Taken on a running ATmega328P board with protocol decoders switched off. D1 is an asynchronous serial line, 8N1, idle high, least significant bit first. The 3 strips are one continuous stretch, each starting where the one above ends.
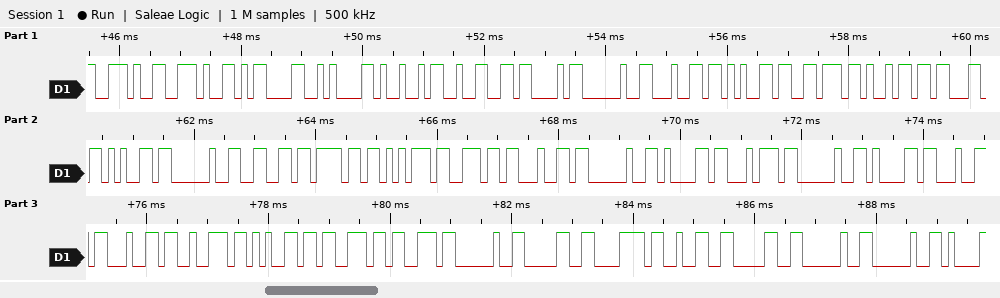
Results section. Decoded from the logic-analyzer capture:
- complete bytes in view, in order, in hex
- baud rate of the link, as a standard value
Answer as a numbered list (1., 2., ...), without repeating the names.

1. 0x2E 0x2E 0x0D 0x0A 0x49 0x32 0x43 0x20 0x64 0x65 0x76 0x69 0x63 0x65 0x20 0x66 0x6F 0x75 0x6E 0x64 0x20 0x61 0x74 0x20 0x61 0x64 0x64 0x72 0x65 0x73 0x73 0x20 0x30 0x78 0x32 0x30 0x20 0x20
2. 9600 baud
